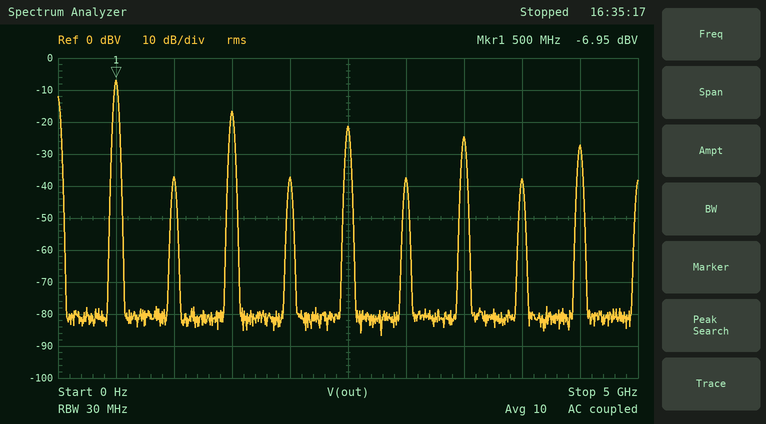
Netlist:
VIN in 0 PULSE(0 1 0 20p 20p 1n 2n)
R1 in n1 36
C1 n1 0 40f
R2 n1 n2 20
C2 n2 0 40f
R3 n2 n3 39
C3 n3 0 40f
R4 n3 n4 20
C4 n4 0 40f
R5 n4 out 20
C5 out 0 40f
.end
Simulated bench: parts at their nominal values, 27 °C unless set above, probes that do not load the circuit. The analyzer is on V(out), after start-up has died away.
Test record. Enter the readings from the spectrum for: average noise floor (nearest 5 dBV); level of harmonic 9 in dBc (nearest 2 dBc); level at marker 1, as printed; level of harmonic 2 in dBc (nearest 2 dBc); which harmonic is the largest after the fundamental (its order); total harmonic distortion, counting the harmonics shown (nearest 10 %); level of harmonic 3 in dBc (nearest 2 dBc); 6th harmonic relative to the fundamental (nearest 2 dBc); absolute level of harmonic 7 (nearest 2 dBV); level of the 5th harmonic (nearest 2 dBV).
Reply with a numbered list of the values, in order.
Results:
1. -80 dBV
2. -20 dBc
3. -6.95 dBV
4. -30 dBc
5. 3
6. 40 %
7. -10 dBc
8. -30 dBc
9. -24 dBV
10. -22 dBV
